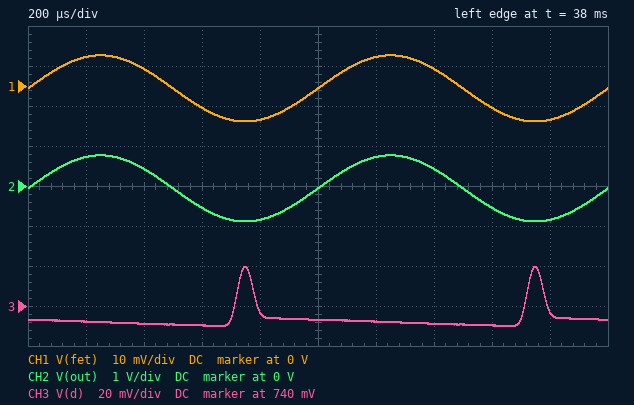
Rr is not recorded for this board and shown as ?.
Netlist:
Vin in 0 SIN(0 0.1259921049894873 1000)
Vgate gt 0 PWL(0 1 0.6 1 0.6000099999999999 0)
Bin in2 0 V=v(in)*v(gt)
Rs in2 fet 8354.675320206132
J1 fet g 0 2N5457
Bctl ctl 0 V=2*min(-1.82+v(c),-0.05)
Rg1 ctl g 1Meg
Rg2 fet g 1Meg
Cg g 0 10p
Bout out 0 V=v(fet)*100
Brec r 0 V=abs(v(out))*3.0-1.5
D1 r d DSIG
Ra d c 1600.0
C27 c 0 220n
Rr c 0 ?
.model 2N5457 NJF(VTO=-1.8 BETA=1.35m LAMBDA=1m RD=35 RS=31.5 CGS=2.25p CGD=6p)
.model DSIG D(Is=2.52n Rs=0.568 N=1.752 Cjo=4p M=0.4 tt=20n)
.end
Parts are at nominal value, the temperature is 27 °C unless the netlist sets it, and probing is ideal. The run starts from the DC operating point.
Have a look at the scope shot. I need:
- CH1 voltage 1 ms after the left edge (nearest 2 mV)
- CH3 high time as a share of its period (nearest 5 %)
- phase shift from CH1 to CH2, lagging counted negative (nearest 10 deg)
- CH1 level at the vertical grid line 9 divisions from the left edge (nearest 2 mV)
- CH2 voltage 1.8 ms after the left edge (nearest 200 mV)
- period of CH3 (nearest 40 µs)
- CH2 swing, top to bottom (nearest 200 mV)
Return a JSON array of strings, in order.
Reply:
["0 V", "5 %", "0 deg", "-8 mV", "-800 mV", "1.00 ms", "1.6 V"]
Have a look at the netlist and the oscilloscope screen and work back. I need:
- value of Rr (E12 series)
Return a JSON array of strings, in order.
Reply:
["680 kΩ"]
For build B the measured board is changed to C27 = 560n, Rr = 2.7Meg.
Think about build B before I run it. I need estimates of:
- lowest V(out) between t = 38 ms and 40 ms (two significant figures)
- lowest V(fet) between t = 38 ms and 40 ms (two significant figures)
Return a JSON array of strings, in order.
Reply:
["-870 mV", "-8.7 mV"]
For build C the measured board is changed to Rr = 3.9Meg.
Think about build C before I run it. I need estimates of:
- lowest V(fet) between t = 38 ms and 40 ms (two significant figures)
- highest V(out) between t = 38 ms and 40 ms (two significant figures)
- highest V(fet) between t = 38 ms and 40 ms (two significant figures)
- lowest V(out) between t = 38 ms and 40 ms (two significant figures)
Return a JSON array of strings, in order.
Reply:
["-8.6 mV", "750 mV", "7.5 mV", "-860 mV"]
